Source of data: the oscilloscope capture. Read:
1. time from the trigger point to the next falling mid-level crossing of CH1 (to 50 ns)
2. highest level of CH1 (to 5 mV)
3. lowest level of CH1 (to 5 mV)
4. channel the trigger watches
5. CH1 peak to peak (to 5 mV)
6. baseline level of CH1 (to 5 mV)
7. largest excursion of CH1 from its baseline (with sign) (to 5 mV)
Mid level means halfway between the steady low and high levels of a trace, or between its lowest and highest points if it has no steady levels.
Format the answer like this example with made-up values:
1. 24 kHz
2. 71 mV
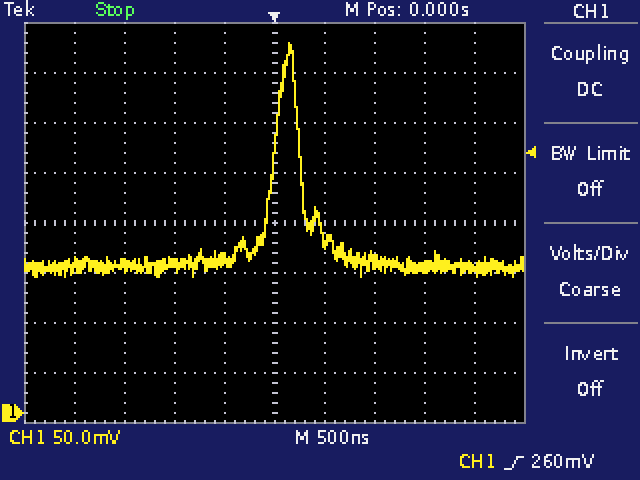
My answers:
1. 250 ns
2. 370 mV
3. 135 mV
4. CH1
5. 235 mV
6. 145 mV
7. +225 mV
